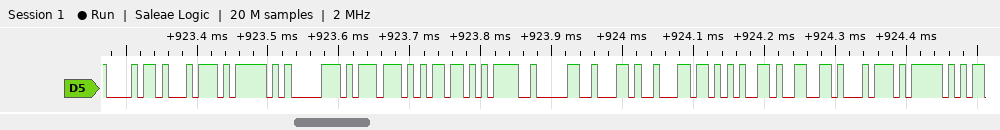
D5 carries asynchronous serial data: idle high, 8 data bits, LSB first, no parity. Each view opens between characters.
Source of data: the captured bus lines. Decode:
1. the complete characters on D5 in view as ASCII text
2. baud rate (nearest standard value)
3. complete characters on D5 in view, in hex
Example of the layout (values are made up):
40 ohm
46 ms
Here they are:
"ht_pwm=0,left_"
115200 baud
68, 74, 5F, 70, 77, 6D, 3D, 30, 2C, 6C, 65, 66, 74, 5F
